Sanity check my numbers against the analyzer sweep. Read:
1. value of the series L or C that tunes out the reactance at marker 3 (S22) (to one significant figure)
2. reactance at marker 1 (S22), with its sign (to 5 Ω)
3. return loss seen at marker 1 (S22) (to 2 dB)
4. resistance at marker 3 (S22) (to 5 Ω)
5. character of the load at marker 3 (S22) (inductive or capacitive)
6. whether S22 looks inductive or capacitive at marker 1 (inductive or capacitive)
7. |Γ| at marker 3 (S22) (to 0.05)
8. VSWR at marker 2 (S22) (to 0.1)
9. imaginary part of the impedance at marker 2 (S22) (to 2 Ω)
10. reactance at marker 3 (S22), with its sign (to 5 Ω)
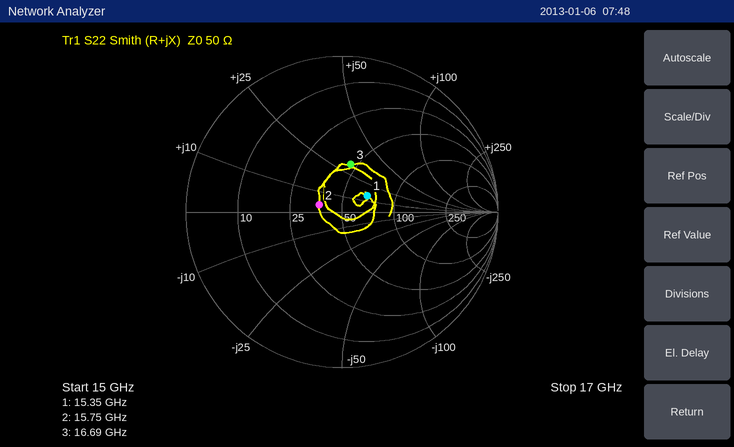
300 fF
+15 Ω
14 dB
45 Ω
inductive
inductive
0.30
1.4
+4 Ω
+30 Ω
